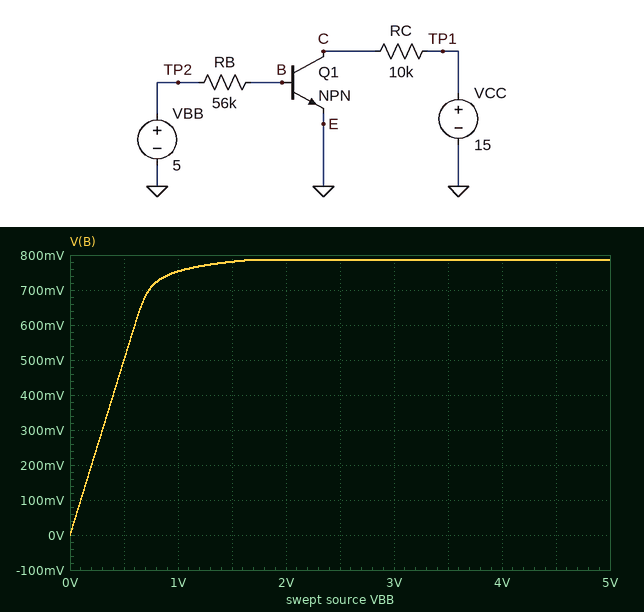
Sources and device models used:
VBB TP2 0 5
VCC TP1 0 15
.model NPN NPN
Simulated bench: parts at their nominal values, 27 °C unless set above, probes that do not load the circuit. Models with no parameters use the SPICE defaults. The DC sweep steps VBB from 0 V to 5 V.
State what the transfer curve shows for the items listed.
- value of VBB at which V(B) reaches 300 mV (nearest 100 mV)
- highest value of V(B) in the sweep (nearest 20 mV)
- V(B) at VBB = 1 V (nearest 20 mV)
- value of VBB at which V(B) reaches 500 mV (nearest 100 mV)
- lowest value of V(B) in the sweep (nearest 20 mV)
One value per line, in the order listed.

300 mV
780 mV
760 mV
500 mV
0 V
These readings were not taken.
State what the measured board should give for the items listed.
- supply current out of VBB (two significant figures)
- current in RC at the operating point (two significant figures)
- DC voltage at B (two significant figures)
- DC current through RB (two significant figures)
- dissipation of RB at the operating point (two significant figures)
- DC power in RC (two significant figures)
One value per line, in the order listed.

75 µA
1.5 mA
790 mV
75 µA
320 µW
22 mW
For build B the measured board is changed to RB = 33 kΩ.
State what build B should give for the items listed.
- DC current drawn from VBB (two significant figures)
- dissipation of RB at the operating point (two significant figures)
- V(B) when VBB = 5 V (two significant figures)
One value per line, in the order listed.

130 µA
540 µW
790 mV
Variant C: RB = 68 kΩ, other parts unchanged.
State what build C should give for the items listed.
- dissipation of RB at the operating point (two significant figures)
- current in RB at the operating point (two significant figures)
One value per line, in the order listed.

260 µW
62 µA
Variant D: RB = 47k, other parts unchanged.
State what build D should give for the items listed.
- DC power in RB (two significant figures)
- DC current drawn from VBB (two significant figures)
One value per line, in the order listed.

380 µW
90 µA
